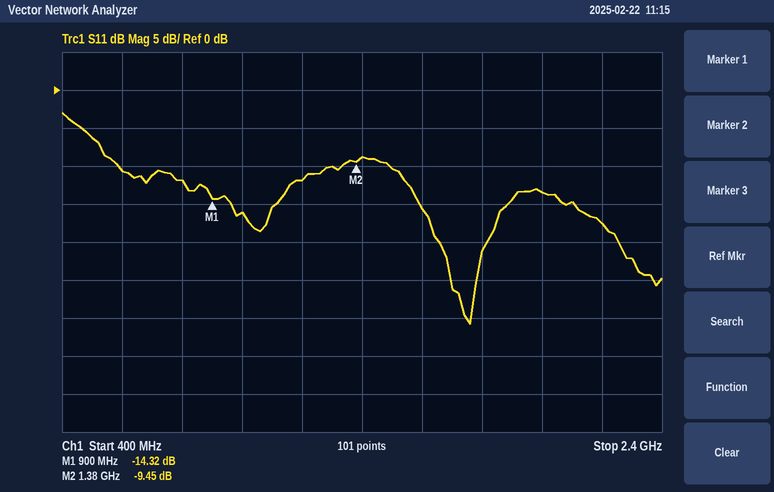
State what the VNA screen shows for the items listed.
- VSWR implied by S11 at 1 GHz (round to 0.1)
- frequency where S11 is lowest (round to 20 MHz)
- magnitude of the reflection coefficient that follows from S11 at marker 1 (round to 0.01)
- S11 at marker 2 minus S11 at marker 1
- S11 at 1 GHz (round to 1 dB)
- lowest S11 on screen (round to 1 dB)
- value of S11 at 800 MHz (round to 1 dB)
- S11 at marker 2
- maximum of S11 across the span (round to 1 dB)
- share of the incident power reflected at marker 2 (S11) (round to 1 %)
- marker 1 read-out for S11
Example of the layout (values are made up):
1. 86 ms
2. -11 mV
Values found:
1. 1.4
2. 1.76 GHz
3. 0.19
4. 4.87 dB
5. -16 dB
6. -31 dB
7. -12 dB
8. -9.45 dB
9. -3 dB
10. 11 %
11. -14.32 dB
